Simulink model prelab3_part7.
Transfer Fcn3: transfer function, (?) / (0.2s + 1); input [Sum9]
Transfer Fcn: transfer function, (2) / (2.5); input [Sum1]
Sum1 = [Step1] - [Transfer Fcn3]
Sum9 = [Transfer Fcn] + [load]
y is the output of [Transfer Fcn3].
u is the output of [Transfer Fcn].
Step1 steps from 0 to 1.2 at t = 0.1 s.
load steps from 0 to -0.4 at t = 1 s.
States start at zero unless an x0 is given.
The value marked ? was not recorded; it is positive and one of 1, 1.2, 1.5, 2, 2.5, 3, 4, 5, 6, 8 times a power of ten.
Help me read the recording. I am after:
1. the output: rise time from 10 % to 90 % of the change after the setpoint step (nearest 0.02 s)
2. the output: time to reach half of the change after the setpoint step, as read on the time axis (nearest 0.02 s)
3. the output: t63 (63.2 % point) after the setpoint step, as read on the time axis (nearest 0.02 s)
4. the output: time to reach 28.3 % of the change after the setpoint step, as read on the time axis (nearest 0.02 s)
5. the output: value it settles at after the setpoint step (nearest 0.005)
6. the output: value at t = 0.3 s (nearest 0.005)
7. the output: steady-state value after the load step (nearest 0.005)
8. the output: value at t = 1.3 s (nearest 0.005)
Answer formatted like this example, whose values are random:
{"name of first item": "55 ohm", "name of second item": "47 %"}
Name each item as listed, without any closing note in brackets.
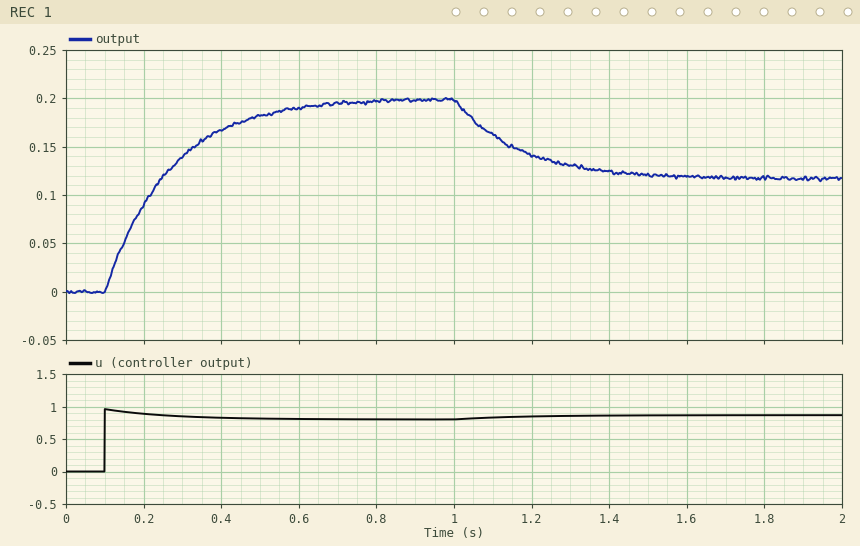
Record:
{"the output: rise time from 10 % to 90 % of the change after the setpoint step": "0.36 s", "the output: time to reach half of the change after the setpoint step, as read on the time axis": "0.22 s", "the output: t63 (63.2 % point) after the setpoint step, as read on the time axis": "0.26 s", "the output: time to reach 28.3 % of the change after the setpoint step, as read on the time axis": "0.16 s", "the output: value it settles at after the setpoint step": "0.200", "the output: value at t = 0.3 s": "0.140", "the output: steady-state value after the load step": "0.115", "the output: value at t = 1.3 s": "0.130"}
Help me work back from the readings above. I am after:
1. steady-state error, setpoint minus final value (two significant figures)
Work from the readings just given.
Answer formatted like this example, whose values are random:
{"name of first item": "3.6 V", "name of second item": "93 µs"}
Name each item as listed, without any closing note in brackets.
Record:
{"steady-state error, setpoint minus final value": "1.0"}
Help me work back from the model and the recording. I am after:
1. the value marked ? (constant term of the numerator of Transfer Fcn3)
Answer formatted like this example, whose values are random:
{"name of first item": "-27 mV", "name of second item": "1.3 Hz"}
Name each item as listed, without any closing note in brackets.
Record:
{"the value marked ?": "0.25"}
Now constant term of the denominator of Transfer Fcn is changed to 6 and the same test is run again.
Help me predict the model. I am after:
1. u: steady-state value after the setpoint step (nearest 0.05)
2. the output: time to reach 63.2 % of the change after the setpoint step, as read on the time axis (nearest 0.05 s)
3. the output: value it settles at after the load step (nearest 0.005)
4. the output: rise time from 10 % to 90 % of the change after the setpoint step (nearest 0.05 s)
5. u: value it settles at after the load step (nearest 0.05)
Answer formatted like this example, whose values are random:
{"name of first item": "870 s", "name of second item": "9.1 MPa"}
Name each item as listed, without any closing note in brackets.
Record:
{"u: steady-state value after the setpoint step": "0.35", "the output: time to reach 63.2 % of the change after the setpoint step, as read on the time axis": "0.30 s", "the output: value it settles at after the load step": "0.000", "the output: rise time from 10 % to 90 % of the change after the setpoint step": "0.40 s", "u: value it settles at after the load step": "0.40"}
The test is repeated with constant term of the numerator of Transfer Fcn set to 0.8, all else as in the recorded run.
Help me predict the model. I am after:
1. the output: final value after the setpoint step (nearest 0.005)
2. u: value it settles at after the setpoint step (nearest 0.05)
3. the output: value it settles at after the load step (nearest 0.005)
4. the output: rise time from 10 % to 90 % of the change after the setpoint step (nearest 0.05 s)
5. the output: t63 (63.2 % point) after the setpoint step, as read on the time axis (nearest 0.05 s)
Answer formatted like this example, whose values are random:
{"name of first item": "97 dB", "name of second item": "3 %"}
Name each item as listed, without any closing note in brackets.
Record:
{"the output: final value after the setpoint step": "0.090", "u: value it settles at after the setpoint step": "0.35", "the output: value it settles at after the load step": "-0.005", "the output: rise time from 10 % to 90 % of the change after the setpoint step": "0.40 s", "the output: t63 (63.2 % point) after the setpoint step, as read on the time axis": "0.30 s"}
